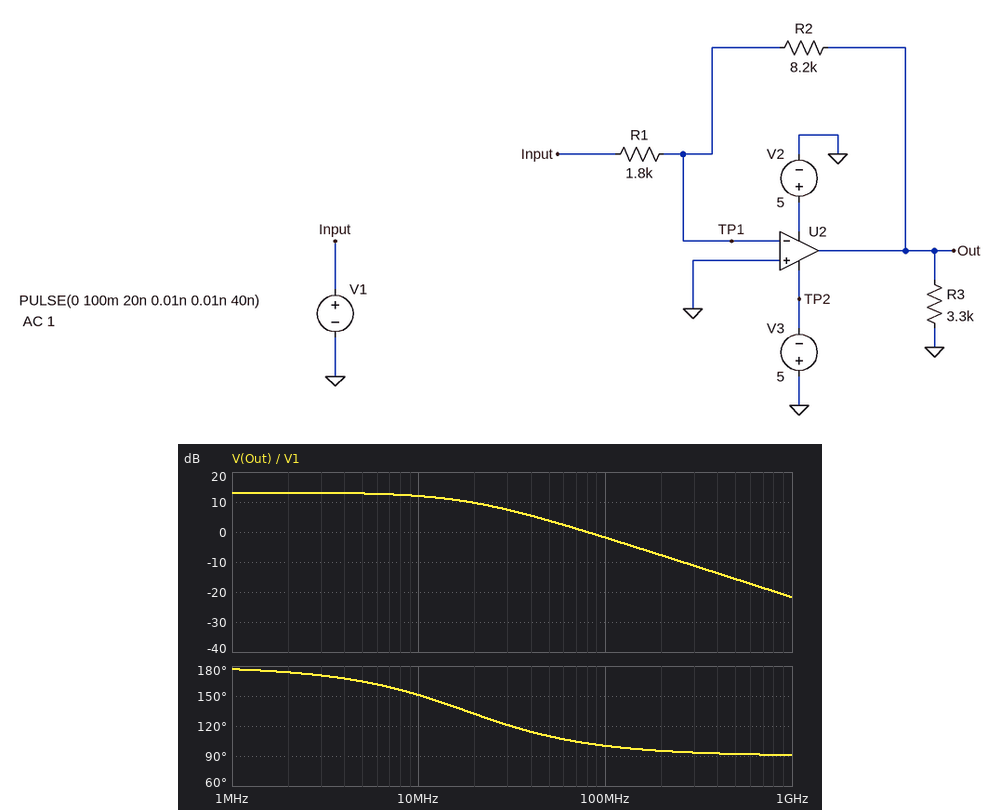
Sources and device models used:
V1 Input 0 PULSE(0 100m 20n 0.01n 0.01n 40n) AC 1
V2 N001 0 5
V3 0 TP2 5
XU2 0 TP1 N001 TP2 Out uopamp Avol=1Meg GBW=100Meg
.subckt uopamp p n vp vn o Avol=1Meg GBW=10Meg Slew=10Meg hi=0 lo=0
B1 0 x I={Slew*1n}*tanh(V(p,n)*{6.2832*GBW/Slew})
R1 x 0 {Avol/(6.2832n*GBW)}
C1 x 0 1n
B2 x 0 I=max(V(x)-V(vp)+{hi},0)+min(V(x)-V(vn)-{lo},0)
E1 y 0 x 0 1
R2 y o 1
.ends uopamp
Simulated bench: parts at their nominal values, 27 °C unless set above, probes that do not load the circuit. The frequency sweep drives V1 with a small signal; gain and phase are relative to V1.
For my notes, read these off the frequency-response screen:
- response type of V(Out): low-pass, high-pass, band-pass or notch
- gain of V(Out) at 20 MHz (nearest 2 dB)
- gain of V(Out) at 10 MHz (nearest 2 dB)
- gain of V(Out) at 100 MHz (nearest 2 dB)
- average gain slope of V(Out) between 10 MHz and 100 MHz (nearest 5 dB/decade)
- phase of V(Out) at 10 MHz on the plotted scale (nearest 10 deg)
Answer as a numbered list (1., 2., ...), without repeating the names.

1. low-pass
2. 10 dB
3. 12 dB
4. -2 dB
5. -15 dB/decade
6. 150 deg
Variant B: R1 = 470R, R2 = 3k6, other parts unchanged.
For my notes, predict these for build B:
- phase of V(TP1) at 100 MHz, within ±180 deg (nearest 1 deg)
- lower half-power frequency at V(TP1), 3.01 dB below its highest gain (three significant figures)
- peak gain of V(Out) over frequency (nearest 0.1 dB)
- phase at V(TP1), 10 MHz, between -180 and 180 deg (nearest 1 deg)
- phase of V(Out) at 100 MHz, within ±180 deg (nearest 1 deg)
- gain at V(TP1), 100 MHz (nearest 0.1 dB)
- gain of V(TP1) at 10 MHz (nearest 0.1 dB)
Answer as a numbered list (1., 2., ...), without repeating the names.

1. 7 deg
2. 11.5 MHz
3. 17.7 dB
4. 49 deg
5. 97 deg
6. -1.1 dB
7. -4.7 dB
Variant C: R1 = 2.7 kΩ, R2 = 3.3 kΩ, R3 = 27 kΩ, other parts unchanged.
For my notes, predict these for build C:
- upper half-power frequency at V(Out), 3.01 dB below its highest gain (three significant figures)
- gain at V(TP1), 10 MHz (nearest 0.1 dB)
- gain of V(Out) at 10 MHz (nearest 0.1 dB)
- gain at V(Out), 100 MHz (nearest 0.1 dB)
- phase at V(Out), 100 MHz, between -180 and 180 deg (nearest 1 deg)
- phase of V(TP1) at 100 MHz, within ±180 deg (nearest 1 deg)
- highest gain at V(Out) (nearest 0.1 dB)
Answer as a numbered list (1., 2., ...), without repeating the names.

1. 45.0 MHz
2. -18.5 dB
3. 1.5 dB
4. -6.0 dB
5. 114 deg
6. 24 deg
7. 1.7 dB
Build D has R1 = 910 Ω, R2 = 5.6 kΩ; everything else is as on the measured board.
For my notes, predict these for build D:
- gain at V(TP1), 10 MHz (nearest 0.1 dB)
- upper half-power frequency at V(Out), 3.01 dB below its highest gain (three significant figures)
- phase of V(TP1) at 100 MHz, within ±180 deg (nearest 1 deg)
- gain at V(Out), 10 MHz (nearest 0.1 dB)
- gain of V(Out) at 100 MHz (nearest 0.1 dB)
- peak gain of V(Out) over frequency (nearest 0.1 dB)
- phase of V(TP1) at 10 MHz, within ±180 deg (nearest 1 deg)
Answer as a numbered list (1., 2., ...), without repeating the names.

1. -6.0 dB
2. 14.0 MHz
3. 8 deg
4. 14.0 dB
5. -1.4 dB
6. 15.8 dB
7. 54 deg
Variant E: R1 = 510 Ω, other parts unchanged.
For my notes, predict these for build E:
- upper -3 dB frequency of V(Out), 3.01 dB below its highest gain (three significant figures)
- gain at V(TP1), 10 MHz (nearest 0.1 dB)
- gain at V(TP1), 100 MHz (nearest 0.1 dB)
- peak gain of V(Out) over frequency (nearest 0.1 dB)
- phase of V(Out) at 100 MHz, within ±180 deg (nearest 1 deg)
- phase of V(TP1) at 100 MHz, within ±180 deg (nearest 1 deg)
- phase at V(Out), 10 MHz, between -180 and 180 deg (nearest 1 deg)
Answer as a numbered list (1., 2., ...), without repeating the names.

1. 5.85 MHz
2. -1.8 dB
3. -0.5 dB
4. 24.1 dB
5. 93 deg
6. 3 deg
7. 120 deg
